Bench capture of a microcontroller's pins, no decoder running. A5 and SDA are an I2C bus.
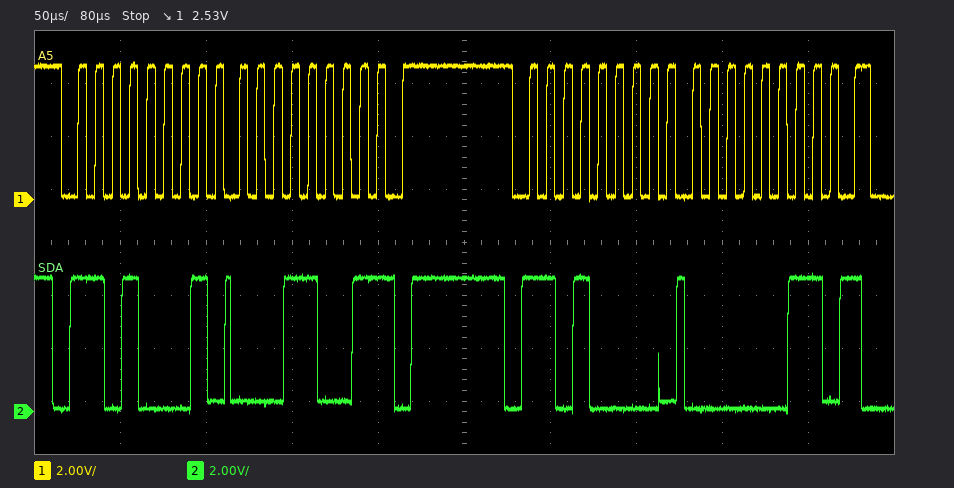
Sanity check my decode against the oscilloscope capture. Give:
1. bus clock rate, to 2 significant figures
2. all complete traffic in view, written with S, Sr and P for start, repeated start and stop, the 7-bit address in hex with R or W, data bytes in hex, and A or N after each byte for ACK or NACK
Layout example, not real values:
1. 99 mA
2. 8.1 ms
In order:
1. 100 kHz
2. S 68R A 19 N P S 68W A 03 A
